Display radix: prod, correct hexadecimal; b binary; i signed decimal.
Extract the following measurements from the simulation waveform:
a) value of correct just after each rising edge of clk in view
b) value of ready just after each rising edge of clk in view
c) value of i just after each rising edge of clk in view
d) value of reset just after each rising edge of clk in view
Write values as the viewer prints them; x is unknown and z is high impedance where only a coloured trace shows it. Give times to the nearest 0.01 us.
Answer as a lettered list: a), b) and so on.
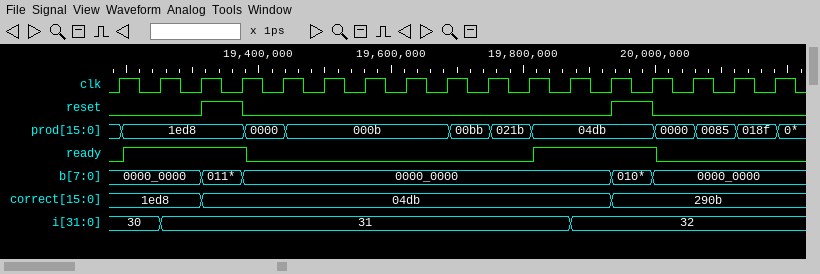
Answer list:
a) 1ed8, 1ed8, 04db, 04db, 04db, 04db, 04db, 04db, 04db, 04db, 04db, 04db, 290b, 290b, 290b, 290b, 290b
b) 0 1 1 1 0 0 0 0 0 0 0 1 1 1 0 0 0
c) 30, 31, 31, 31, 31, 31, 31, 31, 31, 31, 31, 32, 32, 32, 32, 32, 32
d) 0 0 1 0 0 0 0 0 0 0 0 0 1 0 0 0 0
